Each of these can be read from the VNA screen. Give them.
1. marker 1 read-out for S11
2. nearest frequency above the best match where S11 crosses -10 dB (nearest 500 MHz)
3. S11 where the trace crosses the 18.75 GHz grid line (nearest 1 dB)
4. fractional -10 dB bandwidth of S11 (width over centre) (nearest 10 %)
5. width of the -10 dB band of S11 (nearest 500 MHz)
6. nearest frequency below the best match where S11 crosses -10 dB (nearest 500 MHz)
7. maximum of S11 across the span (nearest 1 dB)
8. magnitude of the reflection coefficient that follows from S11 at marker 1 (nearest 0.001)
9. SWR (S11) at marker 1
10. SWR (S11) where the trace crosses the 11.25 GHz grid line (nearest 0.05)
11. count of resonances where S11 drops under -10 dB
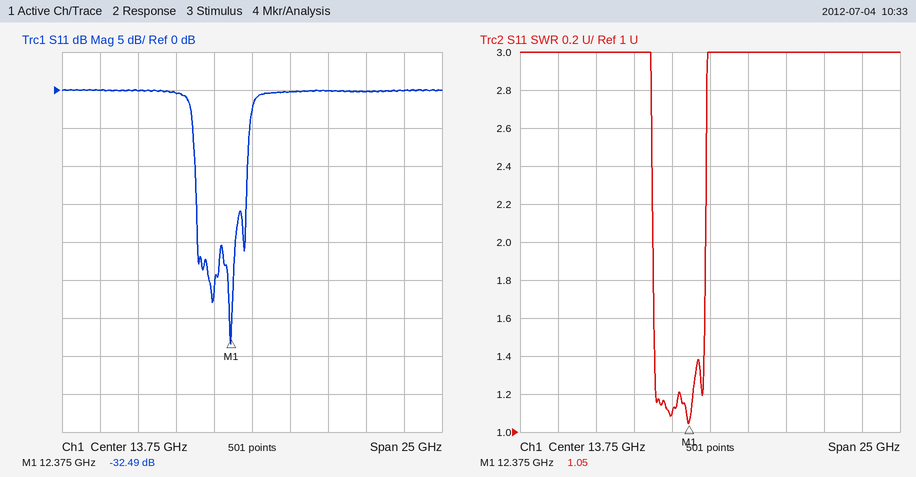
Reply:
-32.49 dB
13.5 GHz
0 dB
30 %
3.5 GHz
10.0 GHz
0 dB
0.024
1.05
1.10
3
